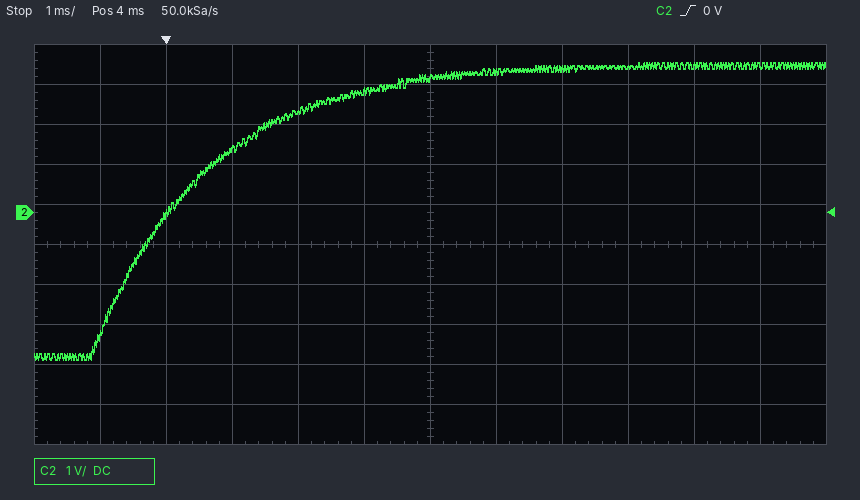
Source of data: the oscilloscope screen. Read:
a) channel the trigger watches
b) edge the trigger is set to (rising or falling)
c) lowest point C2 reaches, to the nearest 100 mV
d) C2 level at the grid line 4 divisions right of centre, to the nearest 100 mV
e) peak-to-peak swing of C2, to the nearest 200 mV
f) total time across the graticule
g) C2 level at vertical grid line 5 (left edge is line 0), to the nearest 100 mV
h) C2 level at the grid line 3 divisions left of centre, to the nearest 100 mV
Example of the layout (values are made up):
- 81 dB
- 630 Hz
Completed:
- C2
- rising
- -3.7 V
- 3.7 V
- 7.4 V
- 12 ms
- 3.0 V
- 1.6 V
